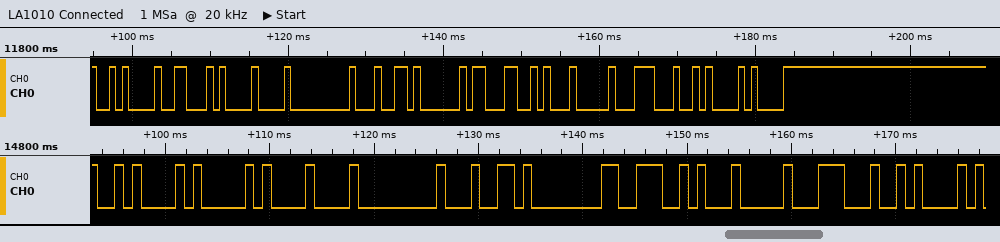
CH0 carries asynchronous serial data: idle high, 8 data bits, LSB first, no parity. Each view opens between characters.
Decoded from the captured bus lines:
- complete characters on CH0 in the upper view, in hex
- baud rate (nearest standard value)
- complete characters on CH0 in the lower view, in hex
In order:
0A, 46, 08, 00, 64, A0, 4C, 04, 1C, 0A, E1
1200 baud
0A, 41, 08, 00, 64, 80, 4E, 04, 1C, 0A
